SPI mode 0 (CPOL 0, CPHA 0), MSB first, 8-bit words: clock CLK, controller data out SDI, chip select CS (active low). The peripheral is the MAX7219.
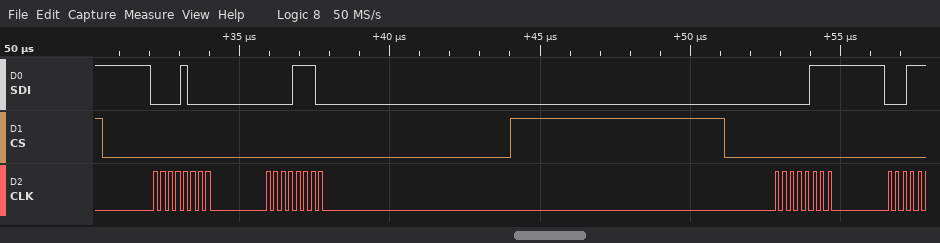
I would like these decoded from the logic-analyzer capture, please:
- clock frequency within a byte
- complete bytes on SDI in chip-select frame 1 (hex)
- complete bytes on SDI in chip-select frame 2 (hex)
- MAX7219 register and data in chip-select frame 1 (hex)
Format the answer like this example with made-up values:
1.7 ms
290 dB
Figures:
4 MHz
08 0E
07
register 0x8, data 0x0E
